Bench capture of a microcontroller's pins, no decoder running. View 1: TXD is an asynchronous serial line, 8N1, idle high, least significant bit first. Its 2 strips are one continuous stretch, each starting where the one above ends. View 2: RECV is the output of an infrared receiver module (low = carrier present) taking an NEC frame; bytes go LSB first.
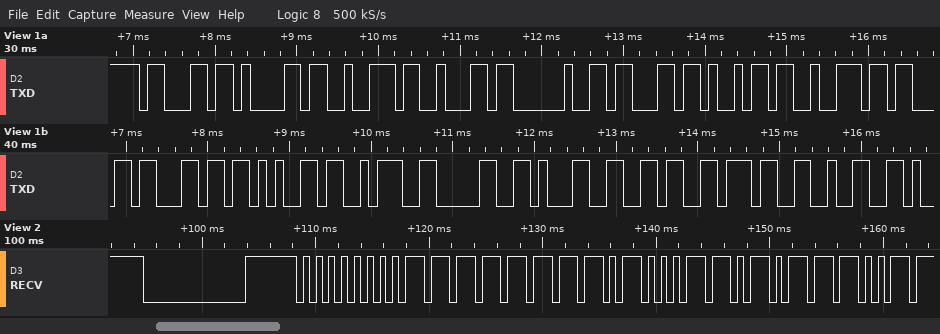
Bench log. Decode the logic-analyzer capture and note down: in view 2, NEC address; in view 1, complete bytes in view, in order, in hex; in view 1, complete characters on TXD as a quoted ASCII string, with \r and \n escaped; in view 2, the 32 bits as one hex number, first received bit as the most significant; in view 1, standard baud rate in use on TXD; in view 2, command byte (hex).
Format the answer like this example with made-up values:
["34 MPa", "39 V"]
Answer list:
["0x00", "63 61 72 62 20 63 69 72 63 6C 65 3A 30 31 36 37 32", "\"carb circle:01672\"", "0x00FF46B9", "9600 baud", "0x62"]
